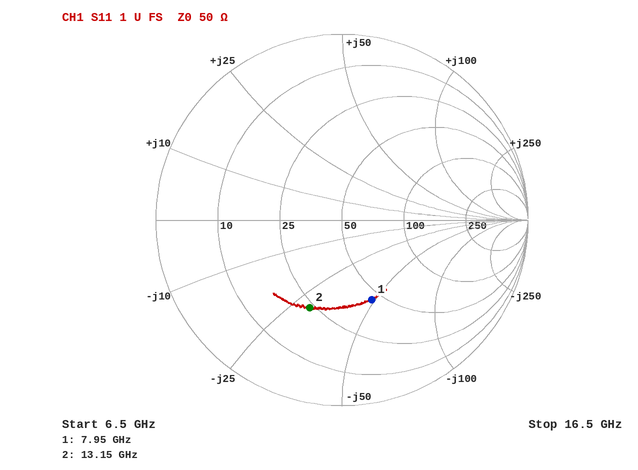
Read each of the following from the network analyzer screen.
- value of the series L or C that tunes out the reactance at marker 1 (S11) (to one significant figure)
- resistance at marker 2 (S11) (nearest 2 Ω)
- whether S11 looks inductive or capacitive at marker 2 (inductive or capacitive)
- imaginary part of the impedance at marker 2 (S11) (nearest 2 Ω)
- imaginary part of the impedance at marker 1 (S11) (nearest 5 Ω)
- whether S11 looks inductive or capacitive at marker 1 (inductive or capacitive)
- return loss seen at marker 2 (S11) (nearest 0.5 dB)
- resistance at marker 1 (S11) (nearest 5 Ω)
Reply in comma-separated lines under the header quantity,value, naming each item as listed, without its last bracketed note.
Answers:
quantity,value
value of the series L or C that tunes out the reactance at marker 1 (S11),1.0 nH
resistance at marker 2 (S11),24 Ω
whether S11 looks inductive or capacitive at marker 2,capacitive
imaginary part of the impedance at marker 2 (S11),-30 Ω
imaginary part of the impedance at marker 1 (S11),-50 Ω
whether S11 looks inductive or capacitive at marker 1,capacitive
return loss seen at marker 2 (S11),6.0 dB
resistance at marker 1 (S11),45 Ω
